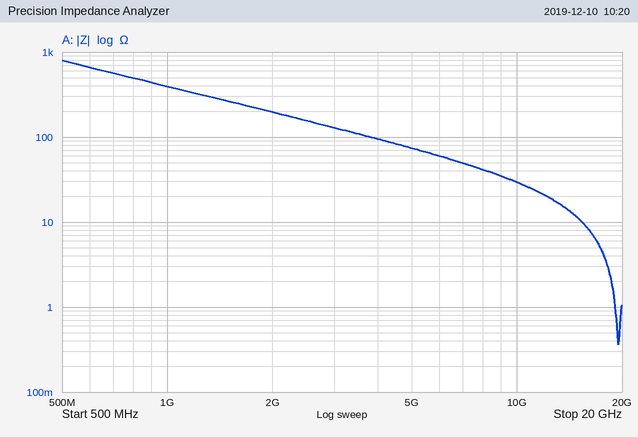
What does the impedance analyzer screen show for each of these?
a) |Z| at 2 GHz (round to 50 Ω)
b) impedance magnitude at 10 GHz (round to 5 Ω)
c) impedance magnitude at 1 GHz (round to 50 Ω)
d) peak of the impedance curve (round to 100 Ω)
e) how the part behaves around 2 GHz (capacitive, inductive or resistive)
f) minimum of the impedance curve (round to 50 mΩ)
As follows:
200 Ω
30 Ω
400 Ω
800 Ω
capacitive
350 mΩ
